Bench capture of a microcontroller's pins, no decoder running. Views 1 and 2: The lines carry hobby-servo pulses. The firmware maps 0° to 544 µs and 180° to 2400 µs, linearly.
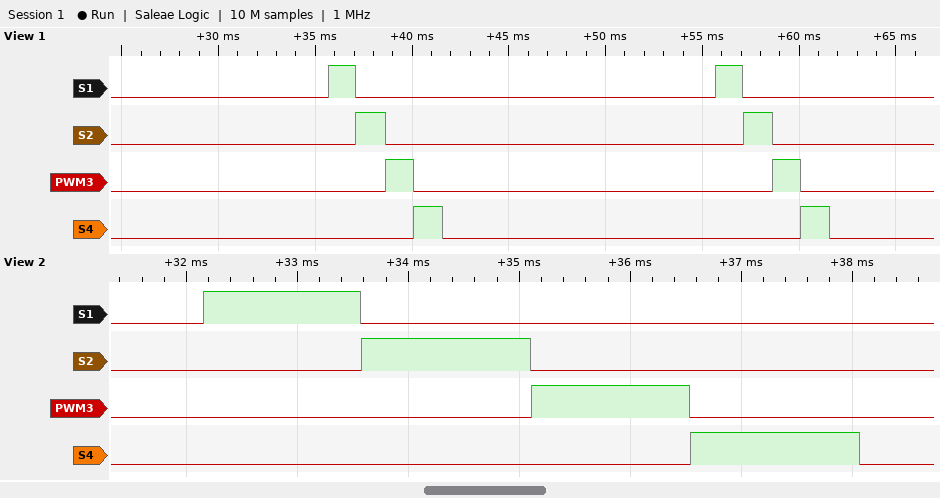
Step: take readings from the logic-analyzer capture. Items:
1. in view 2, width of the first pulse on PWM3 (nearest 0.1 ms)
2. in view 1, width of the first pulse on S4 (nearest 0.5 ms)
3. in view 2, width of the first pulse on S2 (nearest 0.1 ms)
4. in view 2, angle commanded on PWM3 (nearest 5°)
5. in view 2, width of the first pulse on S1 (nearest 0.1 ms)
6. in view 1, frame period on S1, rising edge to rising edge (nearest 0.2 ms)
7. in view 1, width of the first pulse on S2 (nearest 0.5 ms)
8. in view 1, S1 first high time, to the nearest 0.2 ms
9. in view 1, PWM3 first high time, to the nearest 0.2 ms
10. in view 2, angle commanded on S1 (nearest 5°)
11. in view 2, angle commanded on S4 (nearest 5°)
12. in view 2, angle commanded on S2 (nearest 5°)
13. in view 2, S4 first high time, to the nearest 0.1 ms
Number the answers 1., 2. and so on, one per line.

1. 1.4 ms
2. 1.5 ms
3. 1.5 ms
4. 85°
5. 1.4 ms
6. 20.0 ms
7. 1.5 ms
8. 1.4 ms
9. 1.4 ms
10. 85°
11. 95°
12. 95°
13. 1.5 ms
